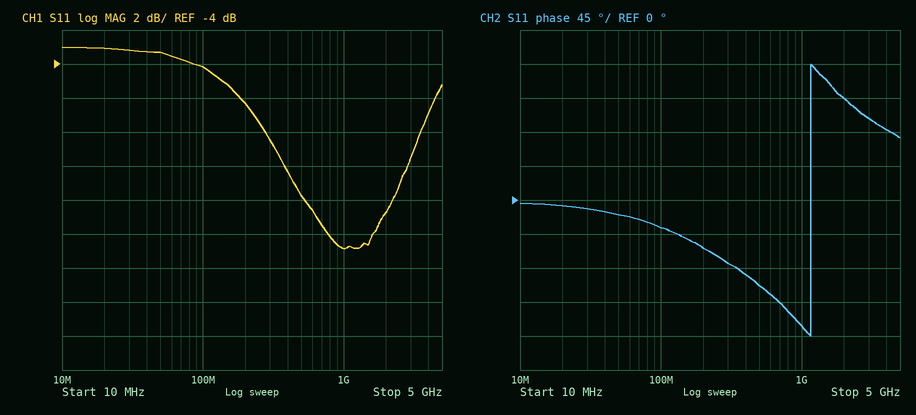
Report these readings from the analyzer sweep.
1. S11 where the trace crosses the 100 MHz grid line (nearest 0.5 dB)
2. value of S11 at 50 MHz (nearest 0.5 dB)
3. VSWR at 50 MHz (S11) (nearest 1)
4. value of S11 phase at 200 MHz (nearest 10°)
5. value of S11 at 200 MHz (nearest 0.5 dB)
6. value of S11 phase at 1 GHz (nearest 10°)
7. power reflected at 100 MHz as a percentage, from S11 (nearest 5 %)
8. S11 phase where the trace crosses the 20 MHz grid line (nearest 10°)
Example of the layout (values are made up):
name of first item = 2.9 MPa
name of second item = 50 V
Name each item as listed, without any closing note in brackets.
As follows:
S11 where the trace crosses the 100 MHz grid line = -4.0 dB
value of S11 at 50 MHz = -3.5 dB
VSWR at 50 MHz (S11) = 5
value of S11 phase at 200 MHz = -60°
value of S11 at 200 MHz = -6.5 dB
value of S11 phase at 1 GHz = -170°
power reflected at 100 MHz as a percentage, from S11 = 40 %
S11 phase where the trace crosses the 20 MHz grid line = -10°
